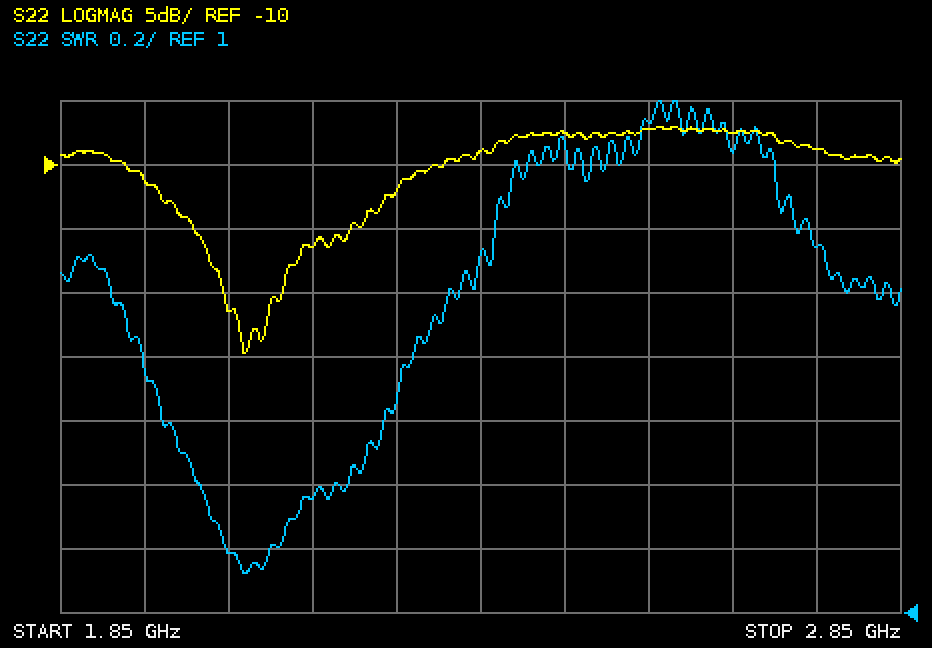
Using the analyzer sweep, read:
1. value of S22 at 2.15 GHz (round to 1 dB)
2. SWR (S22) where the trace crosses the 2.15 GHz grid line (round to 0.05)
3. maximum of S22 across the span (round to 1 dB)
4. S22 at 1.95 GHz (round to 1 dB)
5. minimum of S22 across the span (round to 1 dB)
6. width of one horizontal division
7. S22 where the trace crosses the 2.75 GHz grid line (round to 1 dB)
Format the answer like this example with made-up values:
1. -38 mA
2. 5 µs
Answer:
1. -16 dB
2. 1.35
3. -7 dB
4. -11 dB
5. -25 dB
6. 100 MHz
7. -9 dB
